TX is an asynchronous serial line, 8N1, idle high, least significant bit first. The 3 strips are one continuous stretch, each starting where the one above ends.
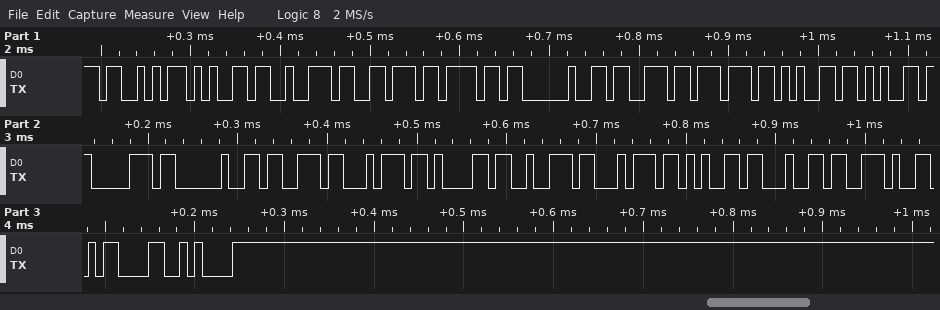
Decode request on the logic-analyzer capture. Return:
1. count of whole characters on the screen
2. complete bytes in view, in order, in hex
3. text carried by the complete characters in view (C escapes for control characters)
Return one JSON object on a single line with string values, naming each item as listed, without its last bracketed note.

{"count of whole characters on the screen": "22", "complete bytes in view, in order, in hex": "0x53 0x65 0x72 0x76 0x6F 0x20 0x73 0x77 0x65 0x65 0x70 0x20 0x73 0x74 0x61 0x72 0x74 0x65 0x64 0x2E 0x0D 0x0A", "text carried by the complete characters in view": "\"Servo sweep started.\\r\\n\""}
